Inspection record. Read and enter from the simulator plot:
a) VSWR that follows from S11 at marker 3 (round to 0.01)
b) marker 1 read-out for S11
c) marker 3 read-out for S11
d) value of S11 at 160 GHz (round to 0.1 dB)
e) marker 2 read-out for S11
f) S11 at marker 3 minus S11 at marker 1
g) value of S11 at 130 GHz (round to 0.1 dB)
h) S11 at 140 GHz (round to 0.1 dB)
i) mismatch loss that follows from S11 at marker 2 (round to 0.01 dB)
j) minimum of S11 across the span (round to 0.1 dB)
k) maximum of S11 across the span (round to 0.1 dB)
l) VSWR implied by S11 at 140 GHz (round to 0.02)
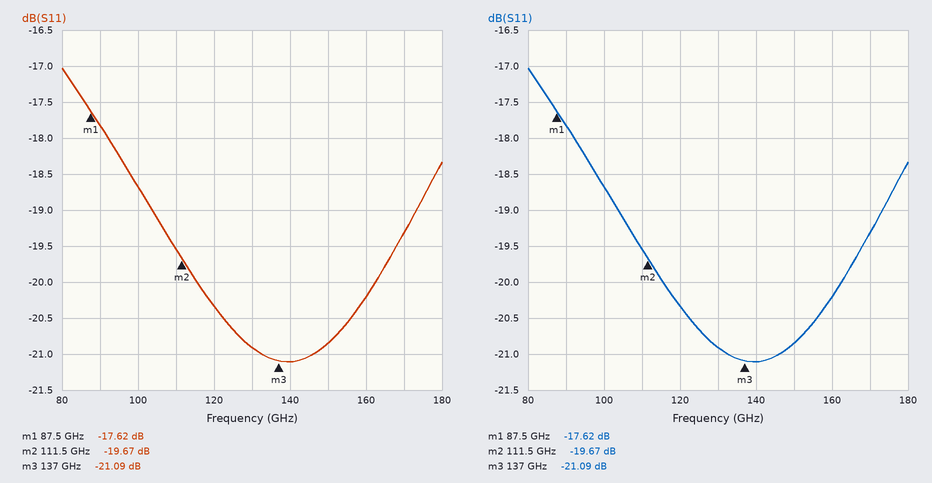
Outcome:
1.19
-17.62 dB
-21.09 dB
-20.2 dB
-19.67 dB
-3.47 dB
-20.9 dB
-21.1 dB
0.05 dB
-21.1 dB
-17.0 dB
1.20
